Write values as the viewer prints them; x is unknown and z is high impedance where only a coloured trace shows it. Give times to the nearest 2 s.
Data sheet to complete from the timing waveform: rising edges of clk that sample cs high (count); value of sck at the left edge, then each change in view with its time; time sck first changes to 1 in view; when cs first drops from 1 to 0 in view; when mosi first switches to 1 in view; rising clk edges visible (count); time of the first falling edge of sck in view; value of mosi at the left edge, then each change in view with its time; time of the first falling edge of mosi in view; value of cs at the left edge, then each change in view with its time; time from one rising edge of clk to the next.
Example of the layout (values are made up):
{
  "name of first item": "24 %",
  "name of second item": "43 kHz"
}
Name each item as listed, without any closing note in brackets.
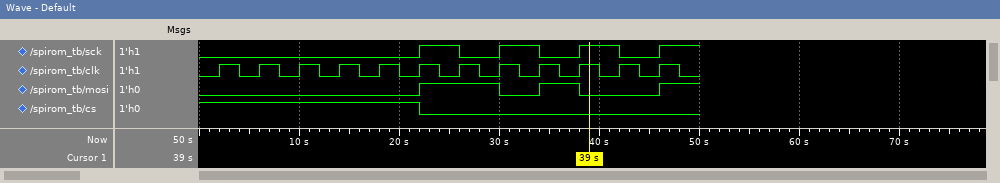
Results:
{
  "rising edges of clk that sample cs high": "6",
  "value of sck at the left edge, then each change in view with its time": "0, 1 at 22 s, 0 at 26 s, 1 at 30 s, 0 at 34 s, 1 at 38 s, 0 at 42 s, 1 at 46 s",
  "time sck first changes to 1 in view": "22 s",
  "when cs first drops from 1 to 0 in view": "22 s",
  "when mosi first switches to 1 in view": "22 s",
  "rising clk edges visible": "12",
  "time of the first falling edge of sck in view": "26 s",
  "value of mosi at the left edge, then each change in view with its time": "0, 1 at 22 s, 0 at 30 s, 1 at 34 s, 0 at 38 s, 1 at 46 s",
  "time of the first falling edge of mosi in view": "30 s",
  "value of cs at the left edge, then each change in view with its time": "1, 0 at 22 s",
  "time from one rising edge of clk to the next": "4 s"
}
